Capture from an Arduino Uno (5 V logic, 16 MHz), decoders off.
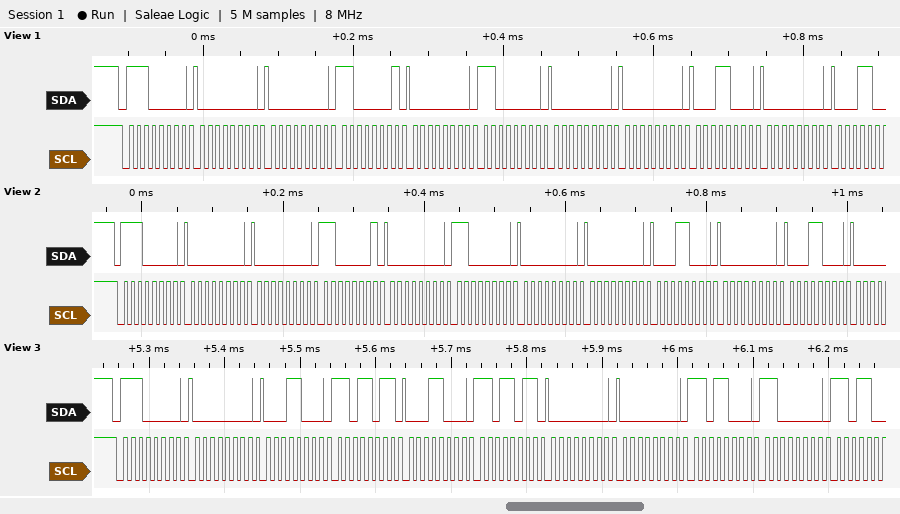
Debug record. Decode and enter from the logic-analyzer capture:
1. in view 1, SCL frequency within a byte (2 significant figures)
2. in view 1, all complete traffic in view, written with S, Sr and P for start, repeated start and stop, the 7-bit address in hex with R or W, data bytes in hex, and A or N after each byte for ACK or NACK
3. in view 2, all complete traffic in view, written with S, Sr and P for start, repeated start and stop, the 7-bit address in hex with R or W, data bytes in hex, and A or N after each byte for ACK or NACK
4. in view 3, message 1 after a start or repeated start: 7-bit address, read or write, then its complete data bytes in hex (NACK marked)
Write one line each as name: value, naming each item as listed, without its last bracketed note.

in view 1, SCL frequency within a byte: 100 kHz
in view 1, all complete traffic in view, written with S, Sr and P for start, repeated start and stop, the 7-bit address in hex with R or W, data bytes in hex, and A or N after each byte for ACK or NACK: S 70W A 00 A 00 A C1 A 00 A C0 A 00 A 00 A 18 A 00 A
in view 2, all complete traffic in view, written with S, Sr and P for start, repeated start and stop, the 7-bit address in hex with R or W, data bytes in hex, and A or N after each byte for ACK or NACK: S 70W A 00 A 00 A C1 A 00 A C0 A 00 A 00 A 18 A 00 A 18 A
in view 3, message 1 after a start or repeated start: 7-bit address, read or write, then its complete data bytes in hex: 0x70 write: 00 18 DB 18 DB 00 00 D8 C0
